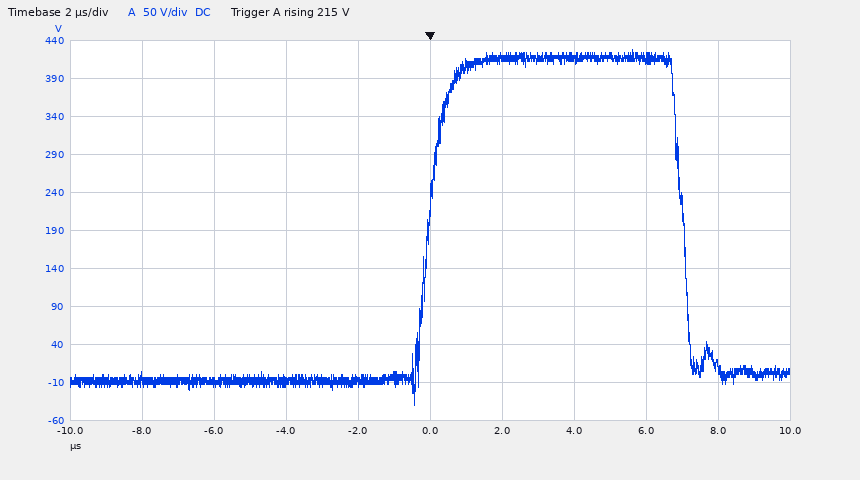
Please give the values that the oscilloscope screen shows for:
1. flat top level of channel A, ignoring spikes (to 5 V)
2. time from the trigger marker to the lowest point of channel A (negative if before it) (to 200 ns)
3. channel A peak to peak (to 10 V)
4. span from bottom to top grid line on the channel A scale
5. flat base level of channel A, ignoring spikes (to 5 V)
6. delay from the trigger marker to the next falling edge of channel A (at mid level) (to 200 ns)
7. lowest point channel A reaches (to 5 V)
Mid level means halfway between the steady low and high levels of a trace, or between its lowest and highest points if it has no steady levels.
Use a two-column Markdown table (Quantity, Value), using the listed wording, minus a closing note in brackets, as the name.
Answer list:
| Quantity | Value |
|---|---|
| flat top level of channel A, ignoring spikes | 415 V |
| time from the trigger marker to the lowest point of channel A (negative if before it) | -400 ns |
| channel A peak to peak | 470 V |
| span from bottom to top grid line on the channel A scale | 500 V |
| flat base level of channel A, ignoring spikes | -10 V |
| delay from the trigger marker to the next falling edge of channel A (at mid level) | 7.0 µs |
| lowest point channel A reaches | -40 V |
